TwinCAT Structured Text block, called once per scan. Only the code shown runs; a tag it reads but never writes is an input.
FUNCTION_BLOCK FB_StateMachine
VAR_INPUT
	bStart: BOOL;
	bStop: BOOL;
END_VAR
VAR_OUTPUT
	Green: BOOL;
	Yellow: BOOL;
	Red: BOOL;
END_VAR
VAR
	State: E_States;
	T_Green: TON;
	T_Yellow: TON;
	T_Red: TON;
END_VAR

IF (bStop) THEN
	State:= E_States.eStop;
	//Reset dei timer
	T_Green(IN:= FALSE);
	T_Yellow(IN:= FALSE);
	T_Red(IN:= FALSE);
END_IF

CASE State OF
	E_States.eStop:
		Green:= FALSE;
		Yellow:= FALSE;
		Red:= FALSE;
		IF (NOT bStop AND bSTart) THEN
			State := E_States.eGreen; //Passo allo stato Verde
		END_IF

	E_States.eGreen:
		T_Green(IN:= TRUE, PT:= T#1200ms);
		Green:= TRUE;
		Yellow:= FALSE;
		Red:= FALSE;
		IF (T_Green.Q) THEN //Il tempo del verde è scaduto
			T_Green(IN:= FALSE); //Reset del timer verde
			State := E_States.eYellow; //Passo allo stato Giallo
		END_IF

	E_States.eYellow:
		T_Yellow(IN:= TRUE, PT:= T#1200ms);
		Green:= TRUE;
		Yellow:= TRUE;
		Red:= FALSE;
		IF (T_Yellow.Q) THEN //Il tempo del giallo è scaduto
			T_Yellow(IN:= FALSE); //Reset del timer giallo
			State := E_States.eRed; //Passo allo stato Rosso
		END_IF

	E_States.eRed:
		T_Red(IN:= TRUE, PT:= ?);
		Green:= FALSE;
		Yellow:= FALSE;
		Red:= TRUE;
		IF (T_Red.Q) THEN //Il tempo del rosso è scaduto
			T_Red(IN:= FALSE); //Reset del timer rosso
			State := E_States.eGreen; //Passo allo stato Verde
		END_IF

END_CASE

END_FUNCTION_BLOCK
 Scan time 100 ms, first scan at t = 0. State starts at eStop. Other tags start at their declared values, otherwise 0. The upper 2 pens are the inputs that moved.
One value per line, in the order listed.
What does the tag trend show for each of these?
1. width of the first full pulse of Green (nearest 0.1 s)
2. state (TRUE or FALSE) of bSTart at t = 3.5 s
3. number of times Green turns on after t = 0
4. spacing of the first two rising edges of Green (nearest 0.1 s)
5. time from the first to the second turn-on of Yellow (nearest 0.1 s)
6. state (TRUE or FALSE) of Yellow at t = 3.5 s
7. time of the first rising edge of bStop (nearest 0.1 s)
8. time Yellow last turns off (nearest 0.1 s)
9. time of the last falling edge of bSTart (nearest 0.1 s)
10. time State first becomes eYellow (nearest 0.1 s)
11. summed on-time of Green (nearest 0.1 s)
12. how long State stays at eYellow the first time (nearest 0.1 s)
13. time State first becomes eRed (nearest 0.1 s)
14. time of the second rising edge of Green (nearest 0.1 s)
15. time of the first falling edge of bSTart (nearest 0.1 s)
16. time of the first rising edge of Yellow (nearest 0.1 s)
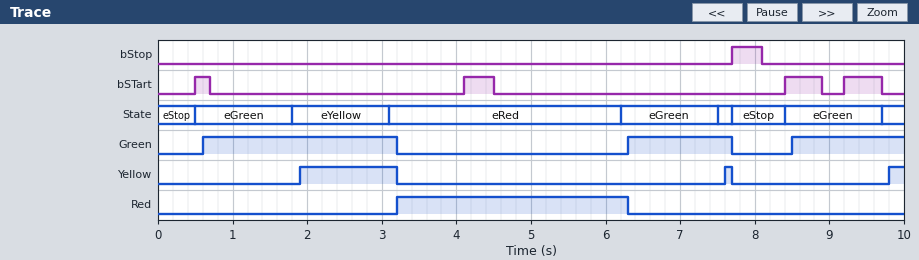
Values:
2.6 s
FALSE
3
5.7 s
5.7 s
FALSE
7.7 s
7.7 s
9.7 s
1.8 s
5.5 s
1.3 s
3.1 s
6.3 s
0.7 s
1.9 s
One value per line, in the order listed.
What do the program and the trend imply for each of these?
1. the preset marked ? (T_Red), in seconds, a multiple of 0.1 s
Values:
3.0 s
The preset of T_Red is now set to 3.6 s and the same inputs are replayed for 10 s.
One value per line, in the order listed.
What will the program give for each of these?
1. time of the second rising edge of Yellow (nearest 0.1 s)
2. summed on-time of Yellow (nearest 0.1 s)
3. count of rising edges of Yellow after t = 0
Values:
9.8 s
1.5 s
2
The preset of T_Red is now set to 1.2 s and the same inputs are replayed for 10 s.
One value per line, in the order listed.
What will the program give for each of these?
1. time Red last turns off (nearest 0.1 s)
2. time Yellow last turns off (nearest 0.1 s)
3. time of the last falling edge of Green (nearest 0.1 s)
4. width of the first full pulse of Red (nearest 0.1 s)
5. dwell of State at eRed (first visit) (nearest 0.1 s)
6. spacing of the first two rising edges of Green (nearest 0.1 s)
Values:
7.7 s
7.1 s
7.1 s
1.3 s
1.3 s
3.9 s
